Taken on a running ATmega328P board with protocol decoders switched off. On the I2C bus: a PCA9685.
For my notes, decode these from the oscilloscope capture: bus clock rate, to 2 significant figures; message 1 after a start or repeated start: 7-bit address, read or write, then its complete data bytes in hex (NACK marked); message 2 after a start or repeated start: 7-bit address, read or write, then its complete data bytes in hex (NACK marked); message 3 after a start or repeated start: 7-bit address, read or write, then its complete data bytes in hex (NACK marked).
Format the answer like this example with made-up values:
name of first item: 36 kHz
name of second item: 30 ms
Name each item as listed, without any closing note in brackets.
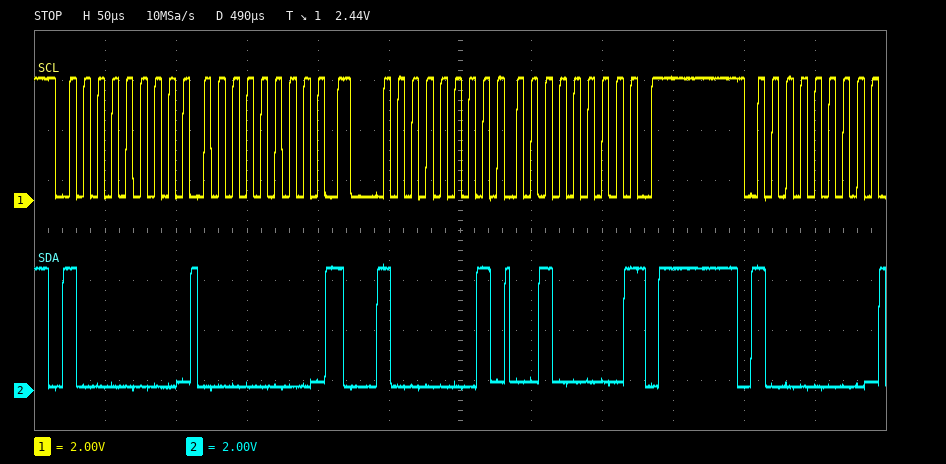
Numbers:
bus clock rate, to 2 significant figures: 100 kHz
message 1 after a start or repeated start: 7-bit address, read or write, then its complete data bytes in hex: 0x40 write: 00
message 2 after a start or repeated start: 7-bit address, read or write, then its complete data bytes in hex: 0x40 read: 20 NACK
message 3 after a start or repeated start: 7-bit address, read or write, then its complete data bytes in hex: 0x40 write
